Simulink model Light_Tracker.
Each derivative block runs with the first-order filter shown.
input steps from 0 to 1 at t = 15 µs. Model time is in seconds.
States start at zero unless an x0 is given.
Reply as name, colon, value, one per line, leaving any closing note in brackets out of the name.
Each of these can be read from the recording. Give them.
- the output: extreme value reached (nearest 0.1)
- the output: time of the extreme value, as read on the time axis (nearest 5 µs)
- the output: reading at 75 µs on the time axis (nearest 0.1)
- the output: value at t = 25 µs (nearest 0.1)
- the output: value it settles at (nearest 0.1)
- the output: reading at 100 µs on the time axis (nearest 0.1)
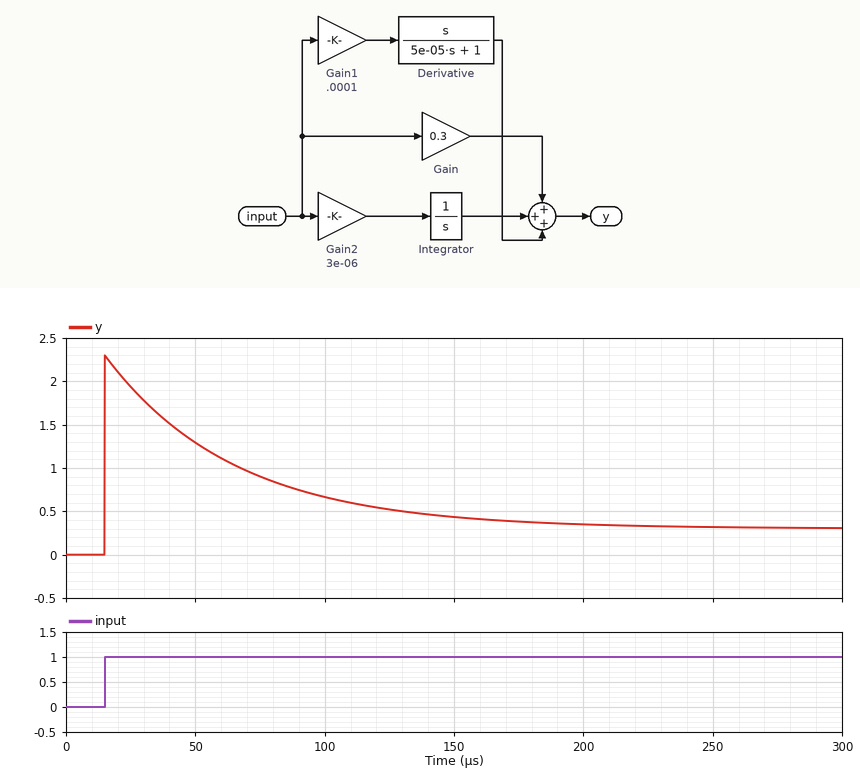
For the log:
the output: extreme value reached: 2.3
the output: time of the extreme value, as read on the time axis: 15 µs
the output: reading at 75 µs on the time axis: 0.9
the output: value at t = 25 µs: 1.9
the output: value it settles at: 0.3
the output: reading at 100 µs on the time axis: 0.7
